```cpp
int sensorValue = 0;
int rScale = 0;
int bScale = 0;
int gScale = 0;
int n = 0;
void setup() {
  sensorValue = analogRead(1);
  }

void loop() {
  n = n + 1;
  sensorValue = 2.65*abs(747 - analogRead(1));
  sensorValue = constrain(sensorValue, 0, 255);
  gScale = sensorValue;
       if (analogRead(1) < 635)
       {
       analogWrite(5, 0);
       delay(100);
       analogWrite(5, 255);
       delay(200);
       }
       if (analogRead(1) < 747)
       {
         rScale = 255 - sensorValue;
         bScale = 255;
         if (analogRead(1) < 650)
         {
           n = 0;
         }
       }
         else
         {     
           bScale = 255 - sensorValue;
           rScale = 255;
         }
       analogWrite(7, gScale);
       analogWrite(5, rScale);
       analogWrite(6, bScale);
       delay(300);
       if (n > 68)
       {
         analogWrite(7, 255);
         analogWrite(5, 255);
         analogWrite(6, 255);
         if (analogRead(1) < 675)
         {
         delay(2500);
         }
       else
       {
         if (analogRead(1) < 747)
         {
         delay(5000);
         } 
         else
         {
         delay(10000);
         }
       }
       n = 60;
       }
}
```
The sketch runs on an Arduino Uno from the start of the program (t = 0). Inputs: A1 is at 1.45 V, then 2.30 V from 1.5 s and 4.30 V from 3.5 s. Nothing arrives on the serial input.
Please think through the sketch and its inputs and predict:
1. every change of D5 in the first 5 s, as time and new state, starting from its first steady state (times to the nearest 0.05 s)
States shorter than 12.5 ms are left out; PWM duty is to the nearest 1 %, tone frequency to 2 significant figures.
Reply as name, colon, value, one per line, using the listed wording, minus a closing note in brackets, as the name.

every change of D5 in the first 5 s, as time and new state, starting from its first steady state: 0 s low; 0.1 s high; 0.3 s low; 0.7 s high; 0.9 s low; 1.3 s high; 1.5 s low; 1.9 s high; 2.1 s low; 2.5 s high; 2.7 s low; 3.1 s high; 3.3 s low; 3.6 s high
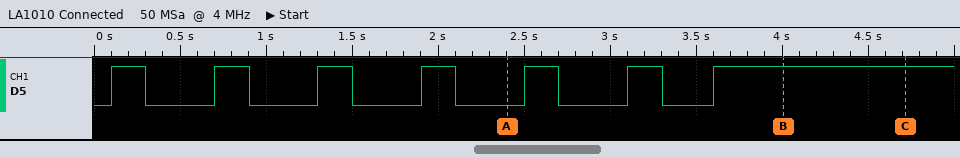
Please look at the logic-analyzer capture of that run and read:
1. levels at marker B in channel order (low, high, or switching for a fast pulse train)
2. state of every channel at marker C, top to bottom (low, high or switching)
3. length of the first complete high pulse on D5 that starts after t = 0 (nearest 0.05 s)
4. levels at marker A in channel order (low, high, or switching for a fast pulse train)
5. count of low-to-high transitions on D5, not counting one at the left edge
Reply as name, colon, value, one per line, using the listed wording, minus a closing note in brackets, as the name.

levels at marker B in channel order: D5 high
state of every channel at marker C, top to bottom: D5 high
length of the first complete high pulse on D5 that starts after t = 0: 0.20 s
levels at marker A in channel order: D5 low
count of low-to-high transitions on D5, not counting one at the left edge: 7
